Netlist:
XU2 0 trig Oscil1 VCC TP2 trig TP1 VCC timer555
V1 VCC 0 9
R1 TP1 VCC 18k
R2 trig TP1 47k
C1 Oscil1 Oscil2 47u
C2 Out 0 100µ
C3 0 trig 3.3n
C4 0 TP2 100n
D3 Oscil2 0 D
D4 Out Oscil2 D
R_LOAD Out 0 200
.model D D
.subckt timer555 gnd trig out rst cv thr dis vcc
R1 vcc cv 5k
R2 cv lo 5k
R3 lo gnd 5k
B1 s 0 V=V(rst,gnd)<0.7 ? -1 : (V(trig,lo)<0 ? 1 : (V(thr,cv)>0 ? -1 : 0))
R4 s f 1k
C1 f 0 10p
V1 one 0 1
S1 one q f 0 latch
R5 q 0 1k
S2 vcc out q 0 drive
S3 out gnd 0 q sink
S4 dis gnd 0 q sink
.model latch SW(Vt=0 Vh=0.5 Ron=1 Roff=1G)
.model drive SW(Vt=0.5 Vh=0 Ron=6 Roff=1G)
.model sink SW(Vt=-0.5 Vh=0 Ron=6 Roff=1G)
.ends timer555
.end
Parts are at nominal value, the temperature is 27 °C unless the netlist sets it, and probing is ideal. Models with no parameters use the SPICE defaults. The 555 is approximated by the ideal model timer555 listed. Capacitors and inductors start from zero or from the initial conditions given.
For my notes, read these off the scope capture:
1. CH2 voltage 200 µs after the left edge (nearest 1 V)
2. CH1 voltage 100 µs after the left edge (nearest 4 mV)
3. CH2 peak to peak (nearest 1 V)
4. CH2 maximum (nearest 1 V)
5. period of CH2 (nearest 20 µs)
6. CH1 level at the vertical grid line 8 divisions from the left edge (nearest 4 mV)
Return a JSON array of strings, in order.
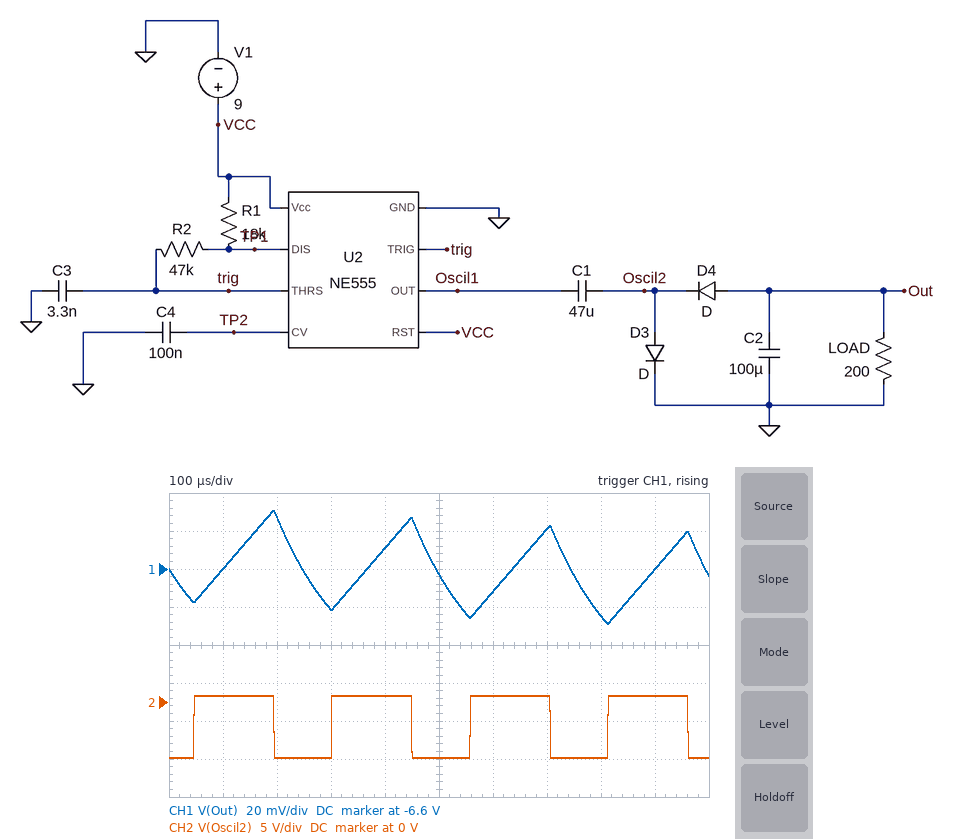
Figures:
["-7 V", "-6.600 V", "8 V", "1 V", "260 µs", "-6.624 V"]
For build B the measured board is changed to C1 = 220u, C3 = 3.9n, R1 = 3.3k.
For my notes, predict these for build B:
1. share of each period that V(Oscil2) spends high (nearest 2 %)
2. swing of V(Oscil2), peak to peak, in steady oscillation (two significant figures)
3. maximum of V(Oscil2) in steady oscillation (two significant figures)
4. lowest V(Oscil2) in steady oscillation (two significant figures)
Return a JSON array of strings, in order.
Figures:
["52 %", "8.0 V", "780 mV", "-7.3 V"]
